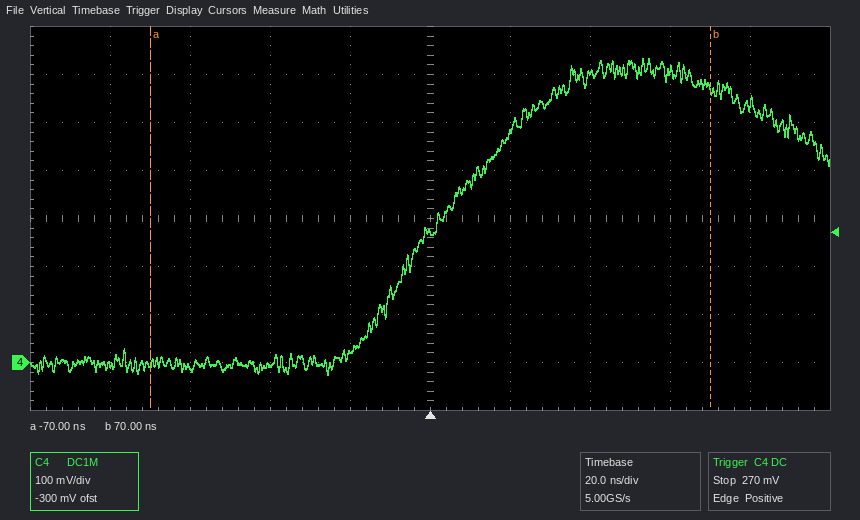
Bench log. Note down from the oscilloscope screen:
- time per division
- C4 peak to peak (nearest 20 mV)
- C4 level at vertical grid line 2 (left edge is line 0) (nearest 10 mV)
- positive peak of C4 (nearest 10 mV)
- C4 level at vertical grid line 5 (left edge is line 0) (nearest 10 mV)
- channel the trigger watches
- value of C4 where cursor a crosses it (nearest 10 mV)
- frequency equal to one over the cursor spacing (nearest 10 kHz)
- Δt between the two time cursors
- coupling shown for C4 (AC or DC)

20 ns
660 mV
-10 mV
630 mV
270 mV
C4
0 mV
7.14 MHz
140 ns
DC
